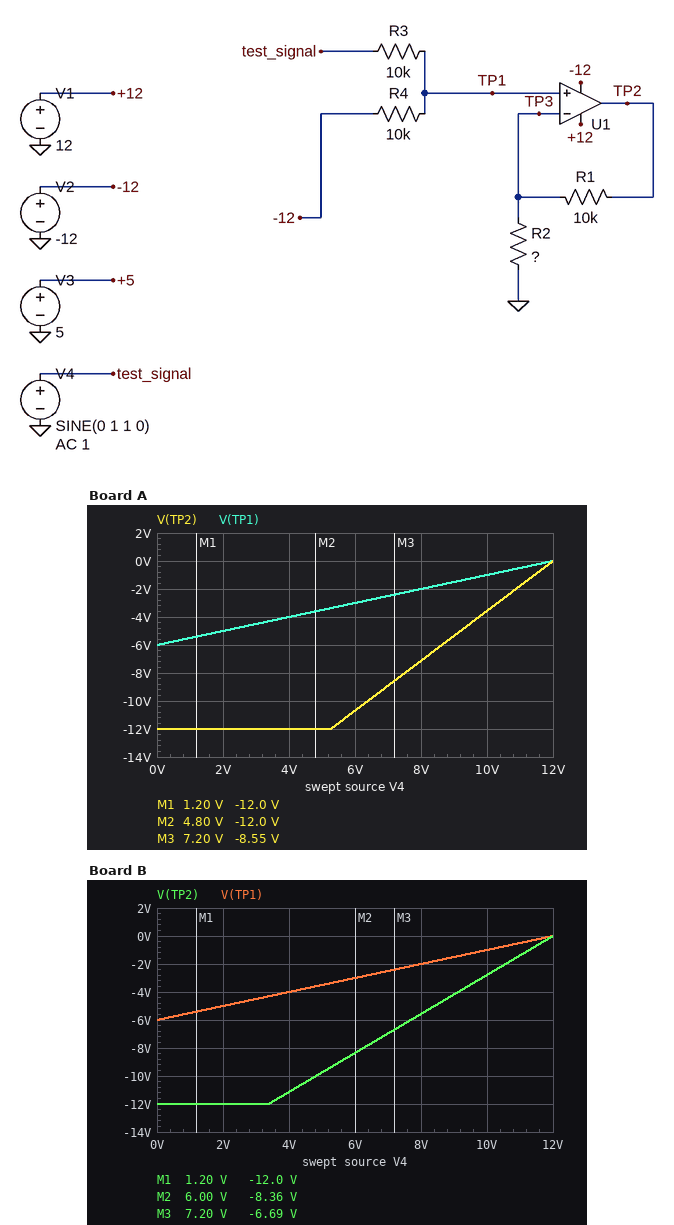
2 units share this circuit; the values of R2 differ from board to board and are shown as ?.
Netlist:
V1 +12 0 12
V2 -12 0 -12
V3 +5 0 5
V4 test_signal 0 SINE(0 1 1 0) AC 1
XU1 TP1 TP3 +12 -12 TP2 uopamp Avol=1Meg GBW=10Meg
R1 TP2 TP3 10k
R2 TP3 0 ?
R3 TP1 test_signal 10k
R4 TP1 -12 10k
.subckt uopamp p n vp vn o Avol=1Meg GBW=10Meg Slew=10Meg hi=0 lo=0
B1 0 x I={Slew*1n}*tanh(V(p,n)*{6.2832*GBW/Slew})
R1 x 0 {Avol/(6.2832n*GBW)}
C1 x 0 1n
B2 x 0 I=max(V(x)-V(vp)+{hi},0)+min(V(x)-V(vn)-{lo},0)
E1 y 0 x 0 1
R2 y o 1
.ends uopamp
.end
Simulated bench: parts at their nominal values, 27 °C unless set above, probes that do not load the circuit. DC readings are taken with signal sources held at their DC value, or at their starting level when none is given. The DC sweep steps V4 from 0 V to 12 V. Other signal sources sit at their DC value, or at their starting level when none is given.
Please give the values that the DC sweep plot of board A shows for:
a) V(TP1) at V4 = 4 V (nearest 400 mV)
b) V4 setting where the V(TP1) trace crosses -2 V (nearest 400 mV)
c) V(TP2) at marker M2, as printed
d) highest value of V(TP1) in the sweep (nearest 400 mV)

-4.0 V
8.0 V
-12.0 V
0 V
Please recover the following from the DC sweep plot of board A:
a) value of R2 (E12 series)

3.9 kΩ
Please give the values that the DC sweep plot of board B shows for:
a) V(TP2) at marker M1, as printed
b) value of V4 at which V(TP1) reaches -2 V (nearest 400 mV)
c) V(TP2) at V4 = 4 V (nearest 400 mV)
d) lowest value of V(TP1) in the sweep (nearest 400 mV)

-12.0 V
8.0 V
-11.2 V
-6.0 V
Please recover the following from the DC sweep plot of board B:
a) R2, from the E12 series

5.6 kΩ
